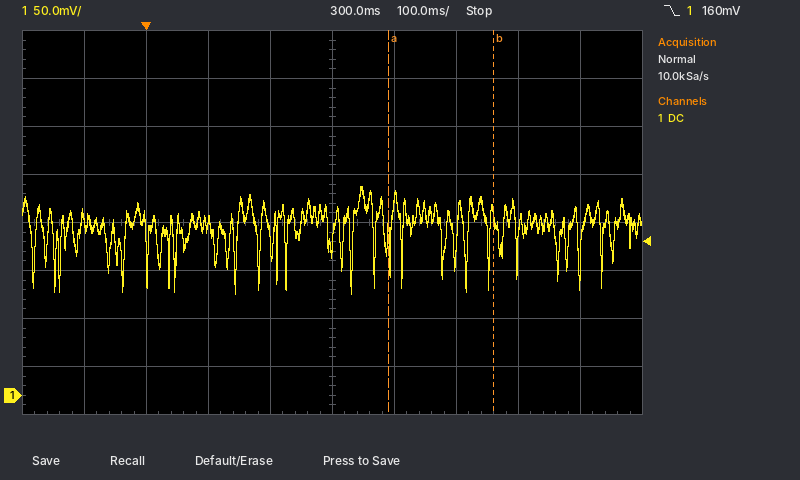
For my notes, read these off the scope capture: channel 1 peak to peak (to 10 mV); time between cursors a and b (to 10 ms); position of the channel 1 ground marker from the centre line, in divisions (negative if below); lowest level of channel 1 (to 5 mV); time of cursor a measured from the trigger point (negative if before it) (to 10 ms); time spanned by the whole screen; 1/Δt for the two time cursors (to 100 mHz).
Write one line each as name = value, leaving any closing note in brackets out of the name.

channel 1 peak to peak = 110 mV
time between cursors a and b = 170 ms
position of the channel 1 ground marker from the centre line, in divisions = -3.6 div
lowest level of channel 1 = 105 mV
time of cursor a measured from the trigger point (negative if before it) = +390 ms
time spanned by the whole screen = 1 s
1/Δt for the two time cursors = 5.9 Hz
